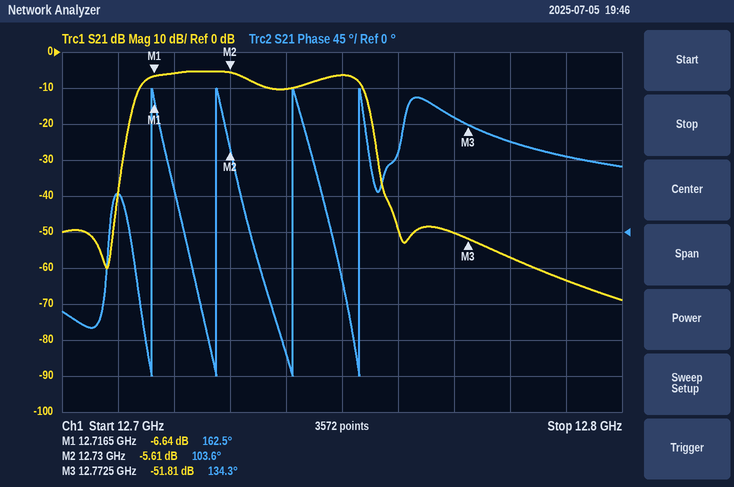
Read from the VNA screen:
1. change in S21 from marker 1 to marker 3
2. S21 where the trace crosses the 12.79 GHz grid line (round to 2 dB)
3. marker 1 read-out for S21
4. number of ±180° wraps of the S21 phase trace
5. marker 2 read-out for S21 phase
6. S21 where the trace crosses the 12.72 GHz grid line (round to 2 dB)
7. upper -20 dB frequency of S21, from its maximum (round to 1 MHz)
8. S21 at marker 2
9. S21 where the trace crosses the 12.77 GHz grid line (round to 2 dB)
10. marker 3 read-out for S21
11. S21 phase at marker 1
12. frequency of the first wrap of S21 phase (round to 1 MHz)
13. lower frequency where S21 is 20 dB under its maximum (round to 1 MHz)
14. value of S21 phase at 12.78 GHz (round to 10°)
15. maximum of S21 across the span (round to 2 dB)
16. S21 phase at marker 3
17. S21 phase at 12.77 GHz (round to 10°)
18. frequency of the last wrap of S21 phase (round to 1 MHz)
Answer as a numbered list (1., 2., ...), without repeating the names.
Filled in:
1. -45.17 dB
2. -64 dB
3. -6.64 dB
4. 4
5. 103.6°
6. -6 dB
7. 12.756 GHz
8. -5.61 dB
9. -50 dB
10. -51.81 dB
11. 162.5°
12. 12.716 GHz
13. 12.711 GHz
14. 110°
15. -6 dB
16. 134.3°
17. 140°
18. 12.753 GHz
